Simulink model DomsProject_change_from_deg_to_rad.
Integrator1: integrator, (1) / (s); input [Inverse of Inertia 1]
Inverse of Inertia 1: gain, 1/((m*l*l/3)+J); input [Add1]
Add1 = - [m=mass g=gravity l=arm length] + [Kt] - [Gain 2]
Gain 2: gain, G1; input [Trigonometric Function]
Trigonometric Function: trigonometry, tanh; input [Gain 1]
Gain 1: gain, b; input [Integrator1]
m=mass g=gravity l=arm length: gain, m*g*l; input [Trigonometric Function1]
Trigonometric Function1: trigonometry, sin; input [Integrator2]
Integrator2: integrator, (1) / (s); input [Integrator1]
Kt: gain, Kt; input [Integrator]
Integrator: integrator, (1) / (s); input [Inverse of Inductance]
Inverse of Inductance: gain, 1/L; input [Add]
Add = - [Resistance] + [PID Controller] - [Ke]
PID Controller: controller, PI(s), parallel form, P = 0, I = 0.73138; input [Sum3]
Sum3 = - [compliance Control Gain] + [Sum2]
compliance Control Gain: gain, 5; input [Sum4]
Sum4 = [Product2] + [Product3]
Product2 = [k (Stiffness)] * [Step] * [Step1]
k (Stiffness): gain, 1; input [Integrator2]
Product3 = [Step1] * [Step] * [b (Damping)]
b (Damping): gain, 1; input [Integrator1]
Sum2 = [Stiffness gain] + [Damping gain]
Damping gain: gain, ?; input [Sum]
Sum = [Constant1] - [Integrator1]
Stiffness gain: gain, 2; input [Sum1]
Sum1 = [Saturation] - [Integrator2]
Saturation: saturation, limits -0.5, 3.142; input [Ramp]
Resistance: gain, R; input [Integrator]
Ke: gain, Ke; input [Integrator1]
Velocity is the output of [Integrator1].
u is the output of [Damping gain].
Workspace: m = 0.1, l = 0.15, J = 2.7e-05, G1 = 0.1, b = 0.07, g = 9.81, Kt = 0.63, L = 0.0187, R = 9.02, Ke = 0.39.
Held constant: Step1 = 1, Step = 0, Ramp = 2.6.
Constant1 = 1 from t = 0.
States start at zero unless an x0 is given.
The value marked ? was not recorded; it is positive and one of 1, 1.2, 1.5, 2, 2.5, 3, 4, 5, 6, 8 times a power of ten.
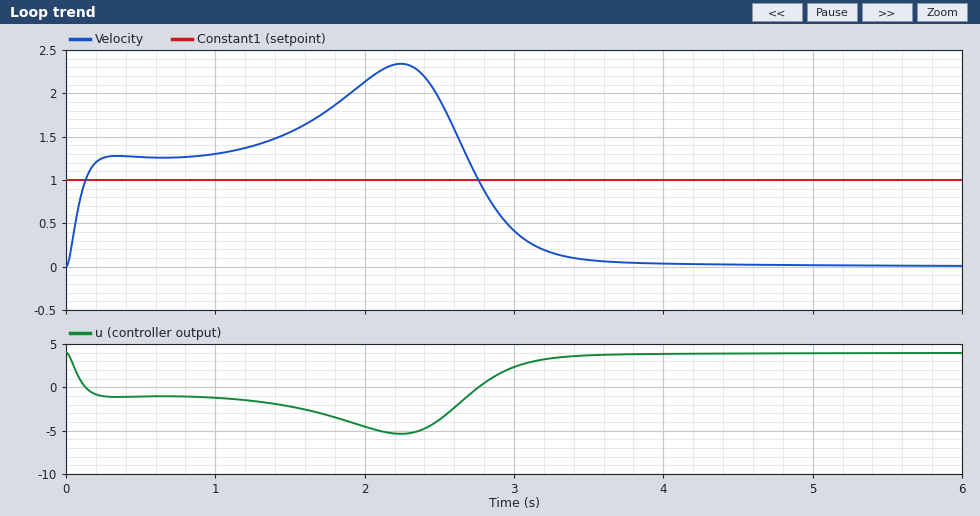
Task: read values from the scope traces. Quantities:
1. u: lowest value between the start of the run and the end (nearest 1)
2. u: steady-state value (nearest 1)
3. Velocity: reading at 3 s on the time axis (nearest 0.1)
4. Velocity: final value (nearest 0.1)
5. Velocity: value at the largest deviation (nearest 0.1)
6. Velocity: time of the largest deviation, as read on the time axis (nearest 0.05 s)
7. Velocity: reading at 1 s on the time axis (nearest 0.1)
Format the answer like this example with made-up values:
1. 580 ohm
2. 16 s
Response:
1. -5
2. 4
3. 0.4
4. 0.0
5. 2.3
6. 2.25 s
7. 1.3
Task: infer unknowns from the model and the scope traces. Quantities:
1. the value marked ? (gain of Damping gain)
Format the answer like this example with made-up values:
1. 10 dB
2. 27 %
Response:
1. 4
